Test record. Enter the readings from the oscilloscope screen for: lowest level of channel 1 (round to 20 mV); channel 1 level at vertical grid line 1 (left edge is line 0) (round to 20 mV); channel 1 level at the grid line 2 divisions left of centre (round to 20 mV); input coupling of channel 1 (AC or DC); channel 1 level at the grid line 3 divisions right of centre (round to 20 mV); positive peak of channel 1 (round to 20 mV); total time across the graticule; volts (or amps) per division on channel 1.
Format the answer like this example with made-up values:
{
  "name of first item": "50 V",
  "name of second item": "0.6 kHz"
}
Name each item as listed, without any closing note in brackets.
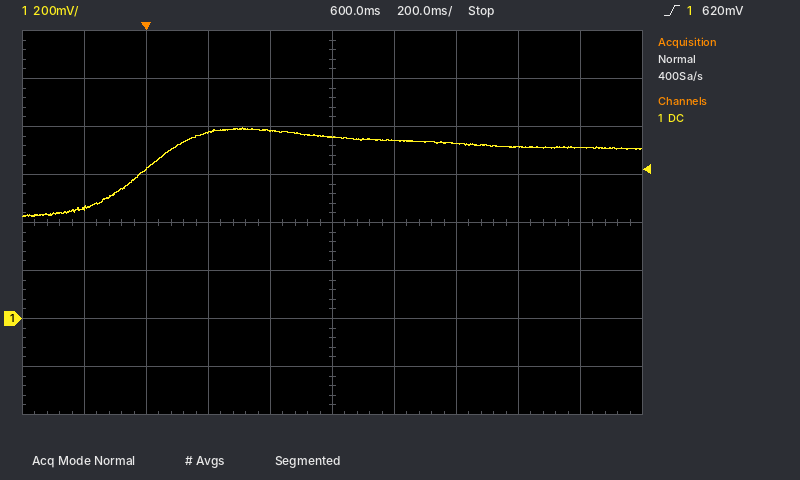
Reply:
{
  "lowest level of channel 1": "420 mV",
  "channel 1 level at vertical grid line 1 (left edge is line 0)": "460 mV",
  "channel 1 level at the grid line 2 divisions left of centre": "780 mV",
  "input coupling of channel 1": "DC",
  "channel 1 level at the grid line 3 divisions right of centre": "720 mV",
  "positive peak of channel 1": "800 mV",
  "total time across the graticule": "2 s",
  "volts (or amps) per division on channel 1": "200 mV"
}
